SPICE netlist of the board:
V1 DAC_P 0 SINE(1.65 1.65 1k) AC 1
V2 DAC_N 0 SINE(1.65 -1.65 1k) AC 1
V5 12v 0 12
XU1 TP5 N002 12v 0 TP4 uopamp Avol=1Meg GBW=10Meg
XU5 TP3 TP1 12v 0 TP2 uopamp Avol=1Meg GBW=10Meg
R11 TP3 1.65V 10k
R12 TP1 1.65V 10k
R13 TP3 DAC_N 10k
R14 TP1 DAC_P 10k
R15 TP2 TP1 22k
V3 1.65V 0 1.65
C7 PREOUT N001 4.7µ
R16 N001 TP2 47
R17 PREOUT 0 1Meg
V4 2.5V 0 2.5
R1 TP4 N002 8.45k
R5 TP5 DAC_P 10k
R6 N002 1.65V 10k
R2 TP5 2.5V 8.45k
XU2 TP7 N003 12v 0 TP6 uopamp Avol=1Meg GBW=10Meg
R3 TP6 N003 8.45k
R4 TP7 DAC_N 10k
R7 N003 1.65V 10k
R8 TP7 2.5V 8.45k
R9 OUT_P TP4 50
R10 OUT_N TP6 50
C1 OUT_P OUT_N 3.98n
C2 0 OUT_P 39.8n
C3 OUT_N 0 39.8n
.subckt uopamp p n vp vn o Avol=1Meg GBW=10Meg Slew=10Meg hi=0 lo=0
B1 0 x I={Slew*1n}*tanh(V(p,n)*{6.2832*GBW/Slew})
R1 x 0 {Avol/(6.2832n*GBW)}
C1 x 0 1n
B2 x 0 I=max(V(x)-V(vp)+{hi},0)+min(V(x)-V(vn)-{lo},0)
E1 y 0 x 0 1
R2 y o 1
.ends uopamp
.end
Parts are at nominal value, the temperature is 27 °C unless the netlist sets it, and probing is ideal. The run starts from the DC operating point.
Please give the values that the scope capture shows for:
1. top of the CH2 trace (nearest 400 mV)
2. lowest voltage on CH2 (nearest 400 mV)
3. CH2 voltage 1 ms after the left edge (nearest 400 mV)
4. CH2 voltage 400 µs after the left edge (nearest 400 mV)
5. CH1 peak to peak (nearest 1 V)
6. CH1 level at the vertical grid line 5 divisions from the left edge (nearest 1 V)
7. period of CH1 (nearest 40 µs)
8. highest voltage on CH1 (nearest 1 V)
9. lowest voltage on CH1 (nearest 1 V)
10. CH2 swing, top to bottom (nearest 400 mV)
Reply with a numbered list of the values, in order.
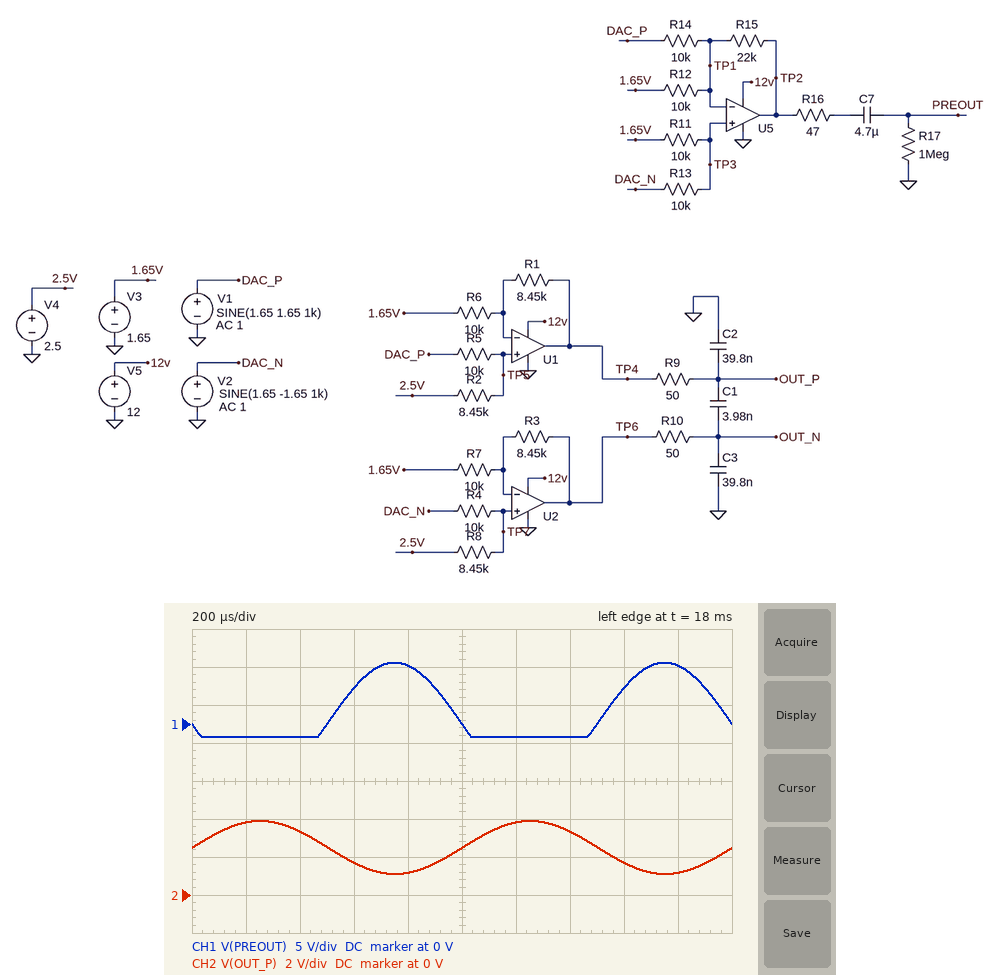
1. 4.0 V
2. 1.2 V
3. 2.4 V
4. 3.2 V
5. 10 V
6. 0 V
7. 1.00 ms
8. 8 V
9. -2 V
10. 2.8 V
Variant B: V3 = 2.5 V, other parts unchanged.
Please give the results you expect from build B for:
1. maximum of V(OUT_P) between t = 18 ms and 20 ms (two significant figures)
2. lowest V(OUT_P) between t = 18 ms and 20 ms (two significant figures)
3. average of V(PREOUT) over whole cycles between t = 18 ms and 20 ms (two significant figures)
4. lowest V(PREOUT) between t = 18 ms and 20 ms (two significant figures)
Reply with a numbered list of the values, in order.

1. 3.2 V
2. 390 mV
3. 1.6 V
4. -2.1 V
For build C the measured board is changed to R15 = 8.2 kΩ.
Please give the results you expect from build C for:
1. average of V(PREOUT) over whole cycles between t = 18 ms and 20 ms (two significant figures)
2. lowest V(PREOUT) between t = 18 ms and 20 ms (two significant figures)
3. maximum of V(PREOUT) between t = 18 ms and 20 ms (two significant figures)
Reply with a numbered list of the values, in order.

1. 420 mV
2. -1.7 V
3. 3.5 V
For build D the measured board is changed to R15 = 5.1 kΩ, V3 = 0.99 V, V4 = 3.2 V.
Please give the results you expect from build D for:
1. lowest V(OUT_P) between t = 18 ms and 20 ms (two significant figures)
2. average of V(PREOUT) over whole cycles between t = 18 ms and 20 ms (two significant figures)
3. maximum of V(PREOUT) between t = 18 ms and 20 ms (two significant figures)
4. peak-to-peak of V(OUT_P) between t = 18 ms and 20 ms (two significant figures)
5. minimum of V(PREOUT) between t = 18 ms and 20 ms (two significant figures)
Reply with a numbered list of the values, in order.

1. 2.4 V
2. 250 mV
3. 2.5 V
4. 2.8 V
5. -1.3 V
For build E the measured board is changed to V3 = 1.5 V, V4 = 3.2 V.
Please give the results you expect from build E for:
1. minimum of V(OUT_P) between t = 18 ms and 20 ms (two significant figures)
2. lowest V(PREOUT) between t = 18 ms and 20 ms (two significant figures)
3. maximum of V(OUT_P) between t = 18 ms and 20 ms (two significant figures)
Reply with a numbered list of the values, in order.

1. 1.9 V
2. -1.6 V
3. 4.7 V
